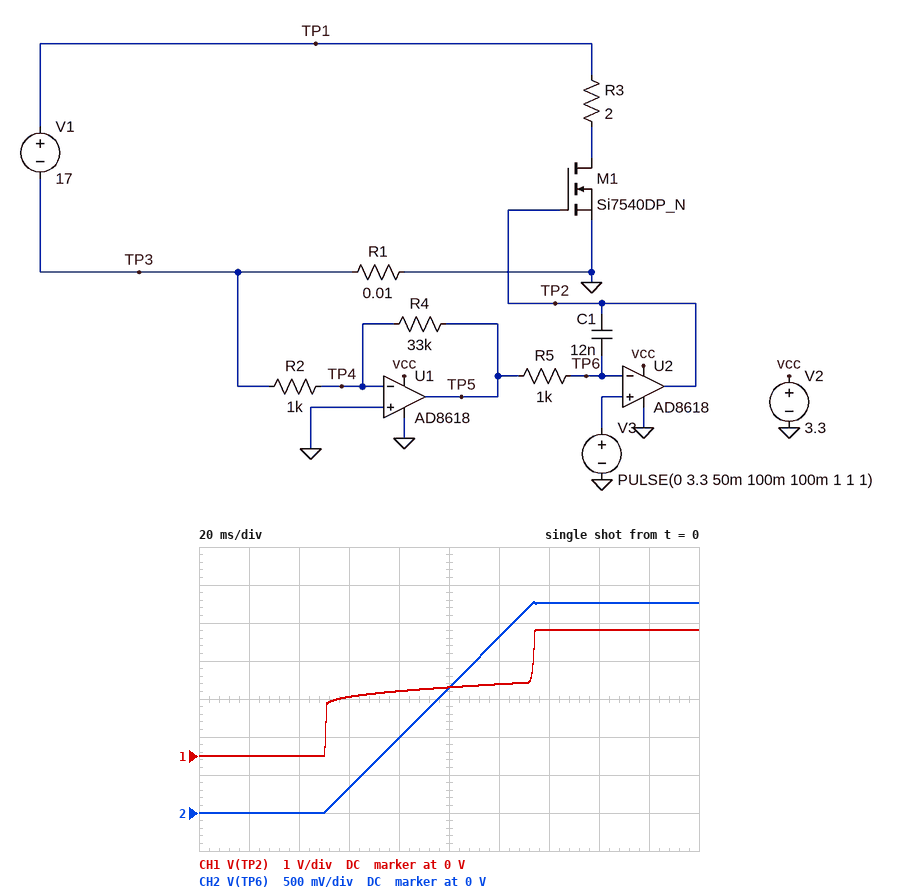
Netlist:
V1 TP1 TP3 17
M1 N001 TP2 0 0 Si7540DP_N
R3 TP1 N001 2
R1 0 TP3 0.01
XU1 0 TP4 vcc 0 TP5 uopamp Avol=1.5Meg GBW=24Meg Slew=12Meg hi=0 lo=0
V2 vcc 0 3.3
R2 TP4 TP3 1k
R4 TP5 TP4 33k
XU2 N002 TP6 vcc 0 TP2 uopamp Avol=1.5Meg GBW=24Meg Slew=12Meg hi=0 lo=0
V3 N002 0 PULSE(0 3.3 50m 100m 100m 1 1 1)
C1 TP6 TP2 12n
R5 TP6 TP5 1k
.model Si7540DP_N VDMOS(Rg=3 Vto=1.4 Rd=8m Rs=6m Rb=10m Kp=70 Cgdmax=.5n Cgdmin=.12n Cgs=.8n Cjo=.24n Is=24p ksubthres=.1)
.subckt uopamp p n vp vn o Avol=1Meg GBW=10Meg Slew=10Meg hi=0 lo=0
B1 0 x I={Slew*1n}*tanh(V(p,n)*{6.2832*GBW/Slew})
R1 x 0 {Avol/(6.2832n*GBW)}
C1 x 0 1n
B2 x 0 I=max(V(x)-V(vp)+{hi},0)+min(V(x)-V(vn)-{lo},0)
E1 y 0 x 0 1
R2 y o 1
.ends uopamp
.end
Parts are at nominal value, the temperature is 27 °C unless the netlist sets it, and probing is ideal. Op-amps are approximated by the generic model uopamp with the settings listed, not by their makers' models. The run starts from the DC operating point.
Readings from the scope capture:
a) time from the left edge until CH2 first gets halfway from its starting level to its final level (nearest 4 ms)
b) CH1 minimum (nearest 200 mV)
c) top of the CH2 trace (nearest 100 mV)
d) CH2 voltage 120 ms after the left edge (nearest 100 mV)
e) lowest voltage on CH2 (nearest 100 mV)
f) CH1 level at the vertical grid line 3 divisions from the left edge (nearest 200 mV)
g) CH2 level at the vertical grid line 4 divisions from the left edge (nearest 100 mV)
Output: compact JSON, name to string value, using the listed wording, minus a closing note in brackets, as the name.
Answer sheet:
{"time from the left edge until CH2 first gets halfway from its starting level to its final level": "92 ms", "CH1 minimum": "0 V", "top of the CH2 trace": "2.8 V", "CH2 voltage 120 ms after the left edge": "2.3 V", "lowest voltage on CH2": "0 V", "CH1 level at the vertical grid line 3 divisions from the left edge": "1.6 V", "CH2 level at the vertical grid line 4 divisions from the left edge": "1.0 V"}
